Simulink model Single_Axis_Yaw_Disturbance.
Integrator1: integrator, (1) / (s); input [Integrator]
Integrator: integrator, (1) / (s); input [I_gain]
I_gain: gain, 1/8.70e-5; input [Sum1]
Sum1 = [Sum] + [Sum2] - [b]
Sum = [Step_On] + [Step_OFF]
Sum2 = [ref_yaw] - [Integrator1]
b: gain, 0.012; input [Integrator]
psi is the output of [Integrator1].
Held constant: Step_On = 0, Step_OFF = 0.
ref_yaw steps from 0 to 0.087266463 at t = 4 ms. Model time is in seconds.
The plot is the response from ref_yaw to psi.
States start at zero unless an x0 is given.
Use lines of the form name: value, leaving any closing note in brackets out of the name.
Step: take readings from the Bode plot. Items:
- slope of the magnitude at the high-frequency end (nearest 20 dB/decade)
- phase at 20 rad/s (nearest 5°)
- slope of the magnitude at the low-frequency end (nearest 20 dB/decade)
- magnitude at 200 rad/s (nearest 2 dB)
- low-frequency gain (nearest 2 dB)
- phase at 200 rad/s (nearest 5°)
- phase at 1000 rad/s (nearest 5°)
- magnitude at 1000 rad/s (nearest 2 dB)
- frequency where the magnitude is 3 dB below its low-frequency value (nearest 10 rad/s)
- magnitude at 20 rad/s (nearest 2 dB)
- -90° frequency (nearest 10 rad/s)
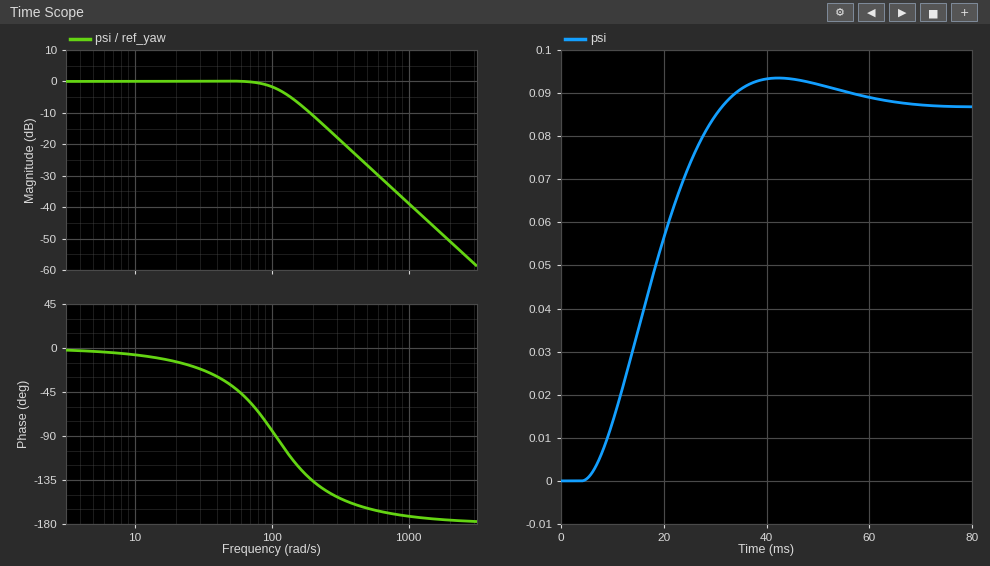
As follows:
slope of the magnitude at the high-frequency end: -40 dB/decade
phase at 20 rad/s: -15°
slope of the magnitude at the low-frequency end: 0 dB/decade
magnitude at 200 rad/s: -10 dB
low-frequency gain: 0 dB
phase at 200 rad/s: -135°
phase at 1000 rad/s: -170°
magnitude at 1000 rad/s: -38 dB
frequency where the magnitude is 3 dB below its low-frequency value: 120 rad/s
magnitude at 20 rad/s: 0 dB
-90° frequency: 110 rad/s
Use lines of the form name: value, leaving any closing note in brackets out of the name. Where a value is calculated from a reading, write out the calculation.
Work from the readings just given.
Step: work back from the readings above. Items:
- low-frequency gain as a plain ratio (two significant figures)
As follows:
low-frequency gain as a plain ratio: 10^(0 / 20) = 1.0
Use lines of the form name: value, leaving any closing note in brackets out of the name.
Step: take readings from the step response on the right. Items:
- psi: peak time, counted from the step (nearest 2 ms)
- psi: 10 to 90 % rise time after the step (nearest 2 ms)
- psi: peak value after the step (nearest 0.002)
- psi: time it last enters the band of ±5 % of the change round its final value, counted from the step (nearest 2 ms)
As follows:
psi: peak time, counted from the step: 38 ms
psi: 10 to 90 % rise time after the step: 18 ms
psi: peak value after the step: 0.094
psi: time it last enters the band of ±5 % of the change round its final value, counted from the step: 48 ms
